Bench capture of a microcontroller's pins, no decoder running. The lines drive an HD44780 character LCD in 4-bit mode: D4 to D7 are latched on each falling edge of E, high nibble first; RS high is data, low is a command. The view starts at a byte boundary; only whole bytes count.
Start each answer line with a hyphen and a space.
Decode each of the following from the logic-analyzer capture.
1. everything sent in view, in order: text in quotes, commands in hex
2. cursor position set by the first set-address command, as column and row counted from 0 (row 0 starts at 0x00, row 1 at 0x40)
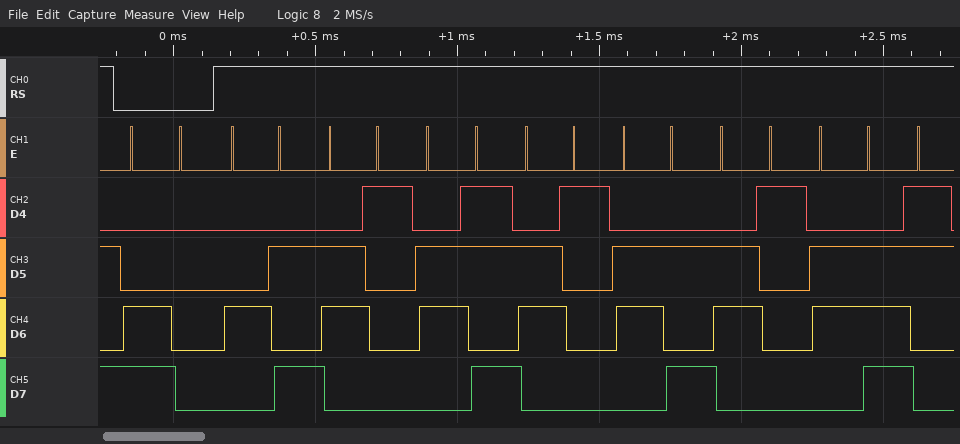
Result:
- 0xC0 "Jakajan"
- column 0, row 1
